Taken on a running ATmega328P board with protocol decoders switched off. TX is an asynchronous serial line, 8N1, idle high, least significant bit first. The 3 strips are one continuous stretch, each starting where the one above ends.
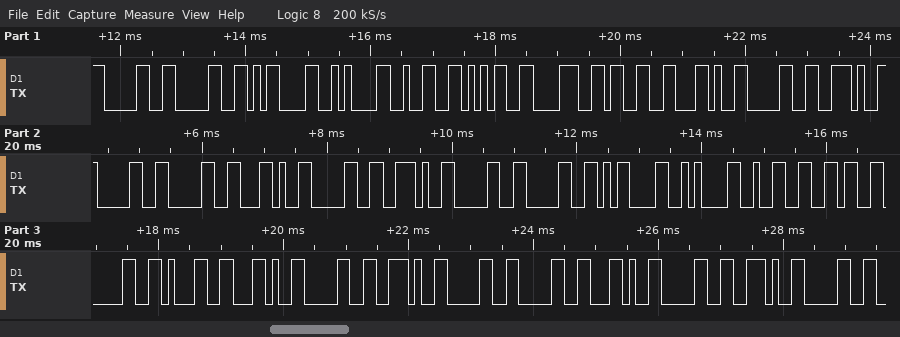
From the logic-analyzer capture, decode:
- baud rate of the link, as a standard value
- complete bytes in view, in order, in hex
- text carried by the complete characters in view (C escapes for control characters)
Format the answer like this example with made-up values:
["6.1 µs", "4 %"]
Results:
["9600 baud", "0x30 0x30 0x0D 0x0A 0x32 0x35 0x38 0x33 0x2C 0x30 0x2E 0x30 0x30 0x2C 0x30 0x2E 0x30 0x30 0x0D 0x0A 0x32 0x36 0x30 0x31 0x2C 0x30 0x2E 0x30 0x30 0x2C 0x30 0x2E 0x30", "\"00\\r\\n2583,0.00,0.00\\r\\n2601,0.00,0.0\""]
